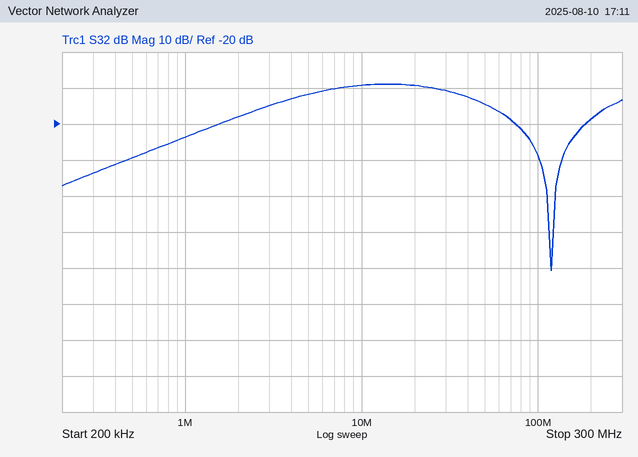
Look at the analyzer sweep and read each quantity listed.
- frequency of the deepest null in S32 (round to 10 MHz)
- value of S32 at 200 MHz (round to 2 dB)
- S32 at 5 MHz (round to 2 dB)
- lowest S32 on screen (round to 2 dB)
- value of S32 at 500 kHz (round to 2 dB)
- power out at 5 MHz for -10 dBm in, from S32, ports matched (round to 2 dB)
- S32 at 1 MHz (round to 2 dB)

120 MHz
-18 dB
-12 dB
-60 dB
-30 dB
-22 dBm
-24 dB
